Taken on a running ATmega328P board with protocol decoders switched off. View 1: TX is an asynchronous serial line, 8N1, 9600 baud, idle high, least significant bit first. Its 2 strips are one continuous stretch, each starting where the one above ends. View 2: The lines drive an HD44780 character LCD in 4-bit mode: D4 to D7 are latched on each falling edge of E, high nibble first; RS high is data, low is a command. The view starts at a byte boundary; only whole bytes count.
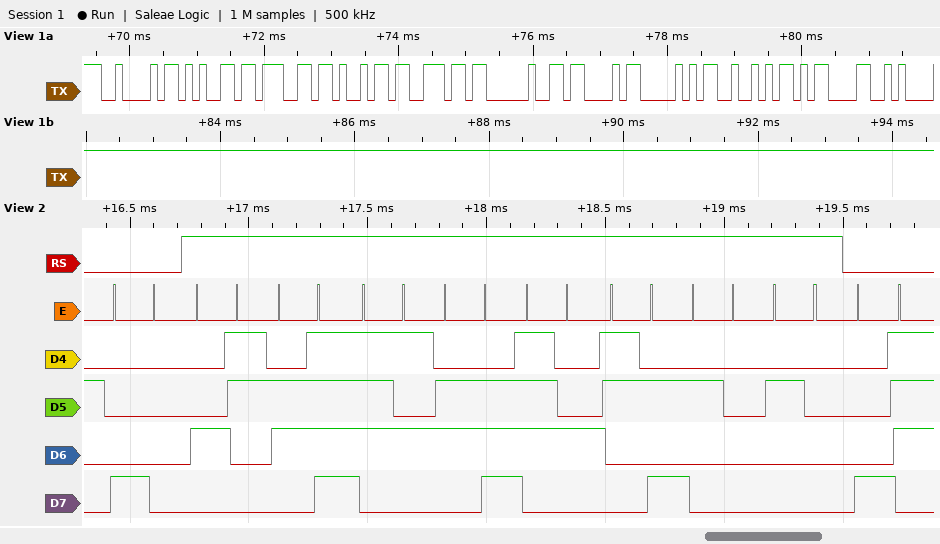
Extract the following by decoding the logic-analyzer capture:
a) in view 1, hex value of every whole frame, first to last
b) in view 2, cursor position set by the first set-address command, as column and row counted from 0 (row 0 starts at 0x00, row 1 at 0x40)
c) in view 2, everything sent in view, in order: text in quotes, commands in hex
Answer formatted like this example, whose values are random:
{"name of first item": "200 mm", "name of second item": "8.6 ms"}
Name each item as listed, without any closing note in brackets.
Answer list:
{"in view 1, hex value of every whole frame, first to last": "42 65 67 69 6E 20 43 50 52 0D 0A", "in view 2, cursor position set by the first set-address command, as column and row counted from 0": "column 0, row 0", "in view 2, everything sent in view, in order: text in quotes, commands in hex": "0x80 \"Count:  \" 0x87"}
